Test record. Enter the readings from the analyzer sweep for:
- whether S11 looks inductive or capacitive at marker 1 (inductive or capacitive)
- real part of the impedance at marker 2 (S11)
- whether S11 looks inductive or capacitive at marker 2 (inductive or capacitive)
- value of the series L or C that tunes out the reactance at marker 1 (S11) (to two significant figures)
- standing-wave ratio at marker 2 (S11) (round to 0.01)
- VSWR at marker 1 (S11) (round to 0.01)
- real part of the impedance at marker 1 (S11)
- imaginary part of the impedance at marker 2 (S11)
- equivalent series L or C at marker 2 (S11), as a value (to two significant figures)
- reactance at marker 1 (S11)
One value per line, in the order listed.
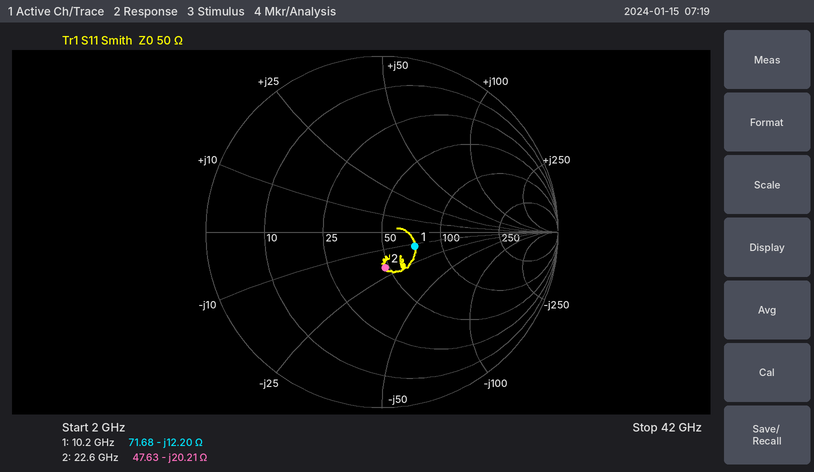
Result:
capacitive
47.63 Ω
capacitive
190 pH
1.51
1.51
71.68 Ω
-20.21 Ω
350 fF
-12.20 Ω
